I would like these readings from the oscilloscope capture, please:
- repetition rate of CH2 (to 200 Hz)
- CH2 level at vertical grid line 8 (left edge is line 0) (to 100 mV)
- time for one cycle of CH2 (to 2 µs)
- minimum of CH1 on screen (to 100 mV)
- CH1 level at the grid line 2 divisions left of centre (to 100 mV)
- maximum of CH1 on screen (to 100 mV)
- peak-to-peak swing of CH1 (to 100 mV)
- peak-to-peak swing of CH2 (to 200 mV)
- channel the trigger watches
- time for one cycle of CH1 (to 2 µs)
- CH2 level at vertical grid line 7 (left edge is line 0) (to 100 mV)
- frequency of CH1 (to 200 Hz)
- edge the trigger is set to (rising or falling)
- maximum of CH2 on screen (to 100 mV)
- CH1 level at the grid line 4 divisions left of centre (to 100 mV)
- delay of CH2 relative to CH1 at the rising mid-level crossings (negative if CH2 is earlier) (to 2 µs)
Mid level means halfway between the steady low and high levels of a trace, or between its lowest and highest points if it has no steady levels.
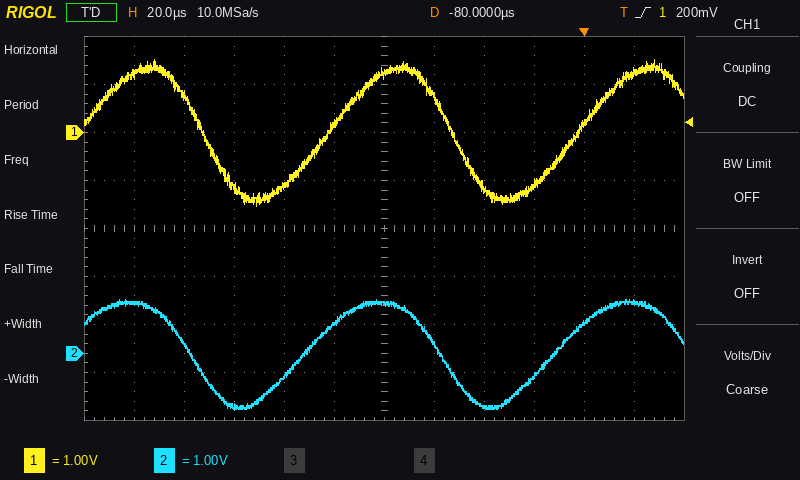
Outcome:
10.0 kHz
-1.1 V
100 µs
-1.5 V
-1.1 V
1.5 V
3.0 V
2.2 V
CH1
100 µs
200 mV
10.0 kHz
rising
1.1 V
800 mV
-10 µs
